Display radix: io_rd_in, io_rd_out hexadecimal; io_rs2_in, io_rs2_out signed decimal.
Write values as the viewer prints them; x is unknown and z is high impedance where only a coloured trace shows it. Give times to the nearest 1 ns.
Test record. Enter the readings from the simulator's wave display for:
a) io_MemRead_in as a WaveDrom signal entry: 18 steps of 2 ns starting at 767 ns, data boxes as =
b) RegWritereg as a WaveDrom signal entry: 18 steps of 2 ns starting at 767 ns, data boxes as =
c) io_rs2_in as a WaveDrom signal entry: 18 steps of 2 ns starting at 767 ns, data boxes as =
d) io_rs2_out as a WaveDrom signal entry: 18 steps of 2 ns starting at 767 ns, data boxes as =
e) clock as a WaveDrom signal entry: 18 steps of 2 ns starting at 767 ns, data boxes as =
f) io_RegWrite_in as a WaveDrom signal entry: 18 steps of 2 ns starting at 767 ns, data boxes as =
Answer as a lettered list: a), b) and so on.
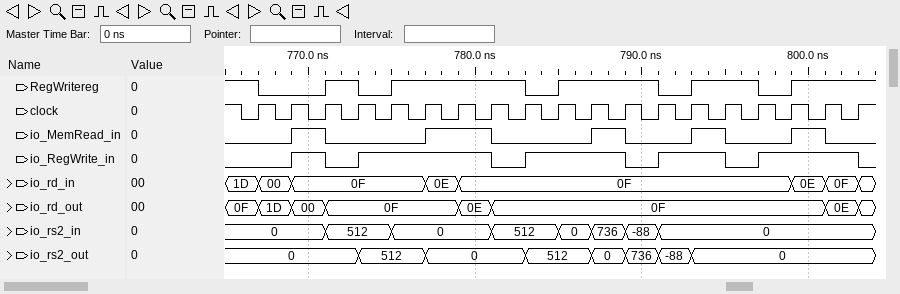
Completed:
a) {name: 'io_MemRead_in', wave: '010..1.0..10.10.10'}
b) {name: 'RegWritereg', wave: '0.101...01..01.01.'}
c) {name: 'io_rs2_in', wave: '=.=.=..=.====.....', data: '0 512 0 512 0 736 -88 0'}
d) {name: 'io_rs2_out', wave: '=..=.=..=.====....', data: '0 512 0 512 0 736 -88 0'}
e) {name: 'clock', wave: 'p.................'}
f) {name: 'io_RegWrite_in', wave: '0101...01..01.01..'}
